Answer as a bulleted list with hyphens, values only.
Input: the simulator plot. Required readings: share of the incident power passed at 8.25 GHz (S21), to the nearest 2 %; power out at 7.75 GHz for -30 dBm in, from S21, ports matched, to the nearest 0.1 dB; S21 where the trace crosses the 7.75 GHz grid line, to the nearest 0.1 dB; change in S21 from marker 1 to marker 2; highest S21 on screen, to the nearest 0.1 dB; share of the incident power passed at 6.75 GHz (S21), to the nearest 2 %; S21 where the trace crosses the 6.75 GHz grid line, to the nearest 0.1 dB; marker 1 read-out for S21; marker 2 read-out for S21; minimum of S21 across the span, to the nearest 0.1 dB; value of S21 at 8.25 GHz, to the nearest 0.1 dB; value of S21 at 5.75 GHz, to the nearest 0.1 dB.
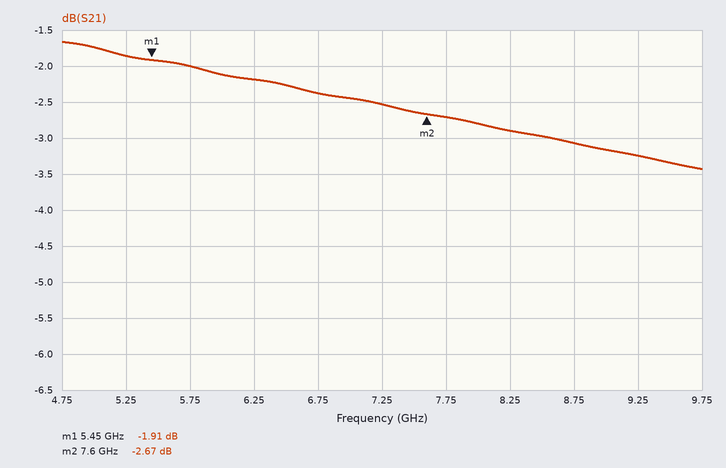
- 52 %
- -32.7 dBm
- -2.7 dB
- -0.76 dB
- -1.7 dB
- 58 %
- -2.4 dB
- -1.91 dB
- -2.67 dB
- -3.4 dB
- -2.9 dB
- -2.0 dB
